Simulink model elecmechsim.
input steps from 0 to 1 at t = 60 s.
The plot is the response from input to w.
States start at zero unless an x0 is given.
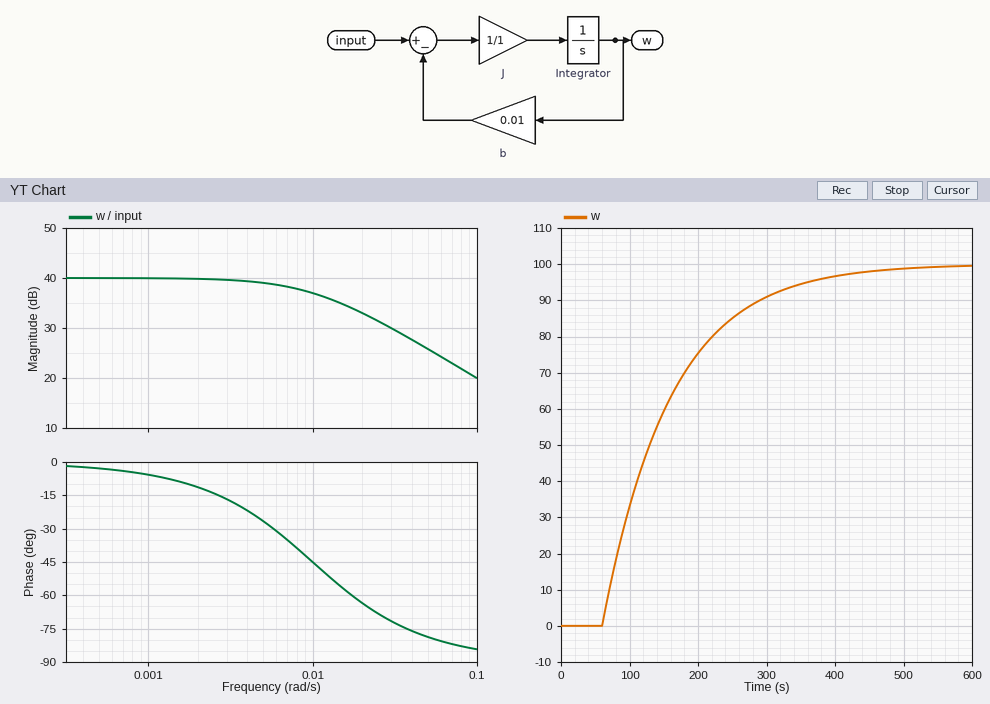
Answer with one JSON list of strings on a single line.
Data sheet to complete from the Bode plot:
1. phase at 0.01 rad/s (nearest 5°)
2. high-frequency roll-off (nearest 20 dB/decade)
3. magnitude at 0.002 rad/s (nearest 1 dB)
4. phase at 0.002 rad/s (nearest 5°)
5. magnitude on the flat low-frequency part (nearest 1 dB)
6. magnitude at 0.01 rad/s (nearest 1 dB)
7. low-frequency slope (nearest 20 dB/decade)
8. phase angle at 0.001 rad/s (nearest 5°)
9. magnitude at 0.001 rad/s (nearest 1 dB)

["-45°", "-20 dB/decade", "40 dB", "-10°", "40 dB", "37 dB", "0 dB/decade", "-5°", "40 dB"]
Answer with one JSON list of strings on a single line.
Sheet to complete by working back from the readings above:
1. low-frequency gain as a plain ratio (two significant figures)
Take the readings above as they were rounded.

["100"]
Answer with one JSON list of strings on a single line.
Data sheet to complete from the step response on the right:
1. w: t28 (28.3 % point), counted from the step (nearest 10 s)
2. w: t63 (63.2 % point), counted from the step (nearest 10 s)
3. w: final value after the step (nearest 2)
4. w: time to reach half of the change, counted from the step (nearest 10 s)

["30 s", "100 s", "100", "70 s"]
